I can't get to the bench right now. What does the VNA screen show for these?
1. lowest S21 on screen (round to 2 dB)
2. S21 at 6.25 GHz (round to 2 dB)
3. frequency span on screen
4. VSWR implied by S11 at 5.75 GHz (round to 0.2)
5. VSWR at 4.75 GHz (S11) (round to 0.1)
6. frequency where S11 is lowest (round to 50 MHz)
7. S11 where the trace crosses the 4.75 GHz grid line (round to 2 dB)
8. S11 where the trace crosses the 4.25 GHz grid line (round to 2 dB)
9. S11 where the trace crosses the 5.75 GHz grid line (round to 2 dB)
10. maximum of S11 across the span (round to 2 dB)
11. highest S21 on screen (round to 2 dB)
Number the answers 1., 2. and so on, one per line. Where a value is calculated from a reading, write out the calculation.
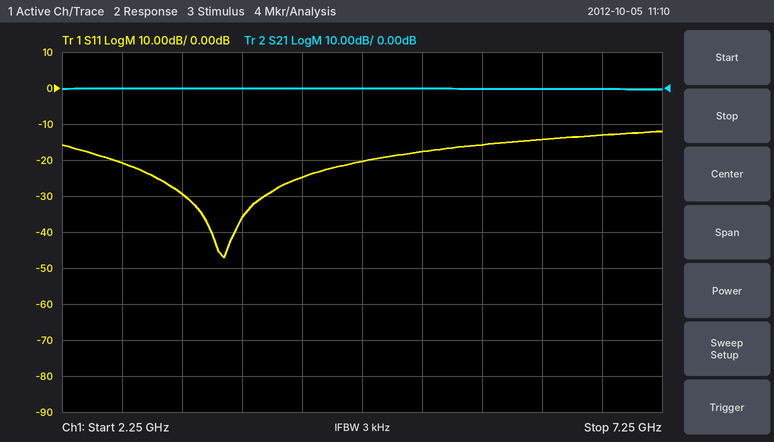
1. 0 dB
2. 0 dB
3. 5 GHz
4. |Γ| = 10^(-16/20) = 0.1585; VSWR = (1 + 0.1585)/(1 − 0.1585) ≈ 1.4
5. |Γ| = 10^(-20/20) = 0.1000; VSWR = (1 + 0.1000)/(1 − 0.1000) ≈ 1.2
6. 3.60 GHz
7. -20 dB
8. -24 dB
9. -16 dB
10. -12 dB
11. 0 dB
